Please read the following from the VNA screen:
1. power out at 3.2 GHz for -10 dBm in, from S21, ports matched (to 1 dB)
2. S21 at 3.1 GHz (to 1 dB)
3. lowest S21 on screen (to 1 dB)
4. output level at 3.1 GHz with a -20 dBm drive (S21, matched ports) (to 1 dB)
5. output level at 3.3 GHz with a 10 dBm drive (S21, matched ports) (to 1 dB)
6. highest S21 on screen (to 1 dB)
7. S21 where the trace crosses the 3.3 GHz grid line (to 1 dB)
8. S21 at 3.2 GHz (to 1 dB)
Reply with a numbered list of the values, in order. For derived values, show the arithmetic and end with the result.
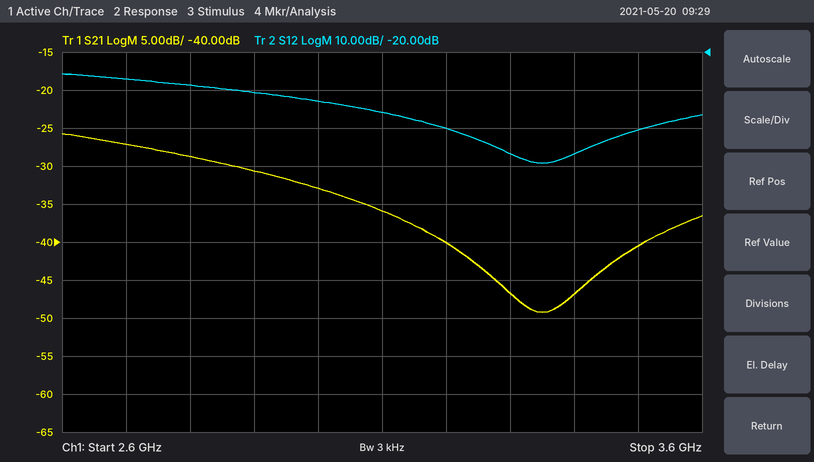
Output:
1. -10 dBm + (-40 dB) = -50 dBm
2. -36 dB
3. -49 dB
4. -20 dBm + (-36 dB) = -56 dBm
5. 10 dBm + (-47 dB) = -37 dBm
6. -26 dB
7. -47 dB
8. -40 dB
